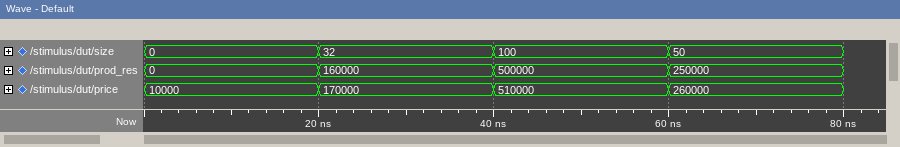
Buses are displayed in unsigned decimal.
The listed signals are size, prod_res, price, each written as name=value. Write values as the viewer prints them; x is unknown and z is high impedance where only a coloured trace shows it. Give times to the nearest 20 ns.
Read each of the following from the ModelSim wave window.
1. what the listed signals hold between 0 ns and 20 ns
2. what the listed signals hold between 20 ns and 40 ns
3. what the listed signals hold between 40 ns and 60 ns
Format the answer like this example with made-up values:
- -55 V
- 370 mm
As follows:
- size=0, prod_res=0, price=10000
- size=32, prod_res=160000, price=170000
- size=100, prod_res=500000, price=510000
